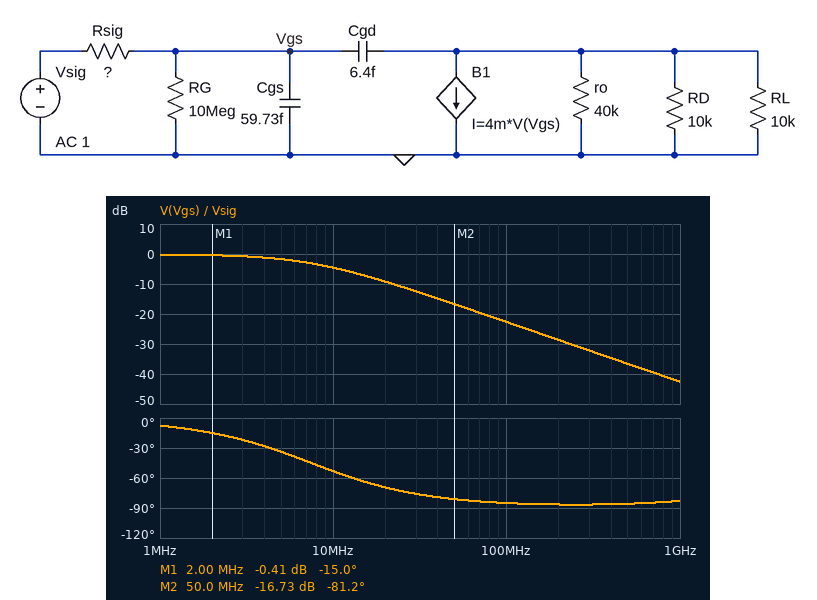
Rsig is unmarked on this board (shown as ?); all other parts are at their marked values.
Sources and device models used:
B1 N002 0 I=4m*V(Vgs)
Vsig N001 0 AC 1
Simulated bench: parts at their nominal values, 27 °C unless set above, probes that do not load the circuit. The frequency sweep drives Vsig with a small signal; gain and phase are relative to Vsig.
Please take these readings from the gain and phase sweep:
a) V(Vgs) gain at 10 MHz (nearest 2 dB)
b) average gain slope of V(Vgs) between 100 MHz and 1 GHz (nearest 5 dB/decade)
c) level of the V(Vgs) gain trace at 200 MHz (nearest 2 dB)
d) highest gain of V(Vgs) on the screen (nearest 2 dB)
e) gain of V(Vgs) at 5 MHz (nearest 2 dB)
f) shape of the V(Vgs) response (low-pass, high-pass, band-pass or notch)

-4 dB
-20 dB/decade
-28 dB
0 dB
-2 dB
low-pass
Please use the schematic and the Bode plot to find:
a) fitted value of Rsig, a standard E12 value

120 kΩ
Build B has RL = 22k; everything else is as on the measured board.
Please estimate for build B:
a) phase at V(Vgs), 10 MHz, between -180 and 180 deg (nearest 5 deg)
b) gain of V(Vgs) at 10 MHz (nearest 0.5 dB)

-60 deg
-5.5 dB
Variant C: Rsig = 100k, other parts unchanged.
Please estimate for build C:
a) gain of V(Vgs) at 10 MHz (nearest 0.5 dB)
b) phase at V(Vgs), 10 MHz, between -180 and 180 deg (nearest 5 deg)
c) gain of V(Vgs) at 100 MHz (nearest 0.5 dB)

-3.5 dB
-50 deg
-21.0 dB
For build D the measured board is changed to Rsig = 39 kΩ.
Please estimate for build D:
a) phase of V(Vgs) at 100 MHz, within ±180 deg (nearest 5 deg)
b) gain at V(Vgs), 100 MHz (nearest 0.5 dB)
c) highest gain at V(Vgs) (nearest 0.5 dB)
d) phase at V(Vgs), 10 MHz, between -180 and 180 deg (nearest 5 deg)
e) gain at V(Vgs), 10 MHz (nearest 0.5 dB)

-75 deg
-13.0 dB
0 dB
-25 deg
-1.0 dB
